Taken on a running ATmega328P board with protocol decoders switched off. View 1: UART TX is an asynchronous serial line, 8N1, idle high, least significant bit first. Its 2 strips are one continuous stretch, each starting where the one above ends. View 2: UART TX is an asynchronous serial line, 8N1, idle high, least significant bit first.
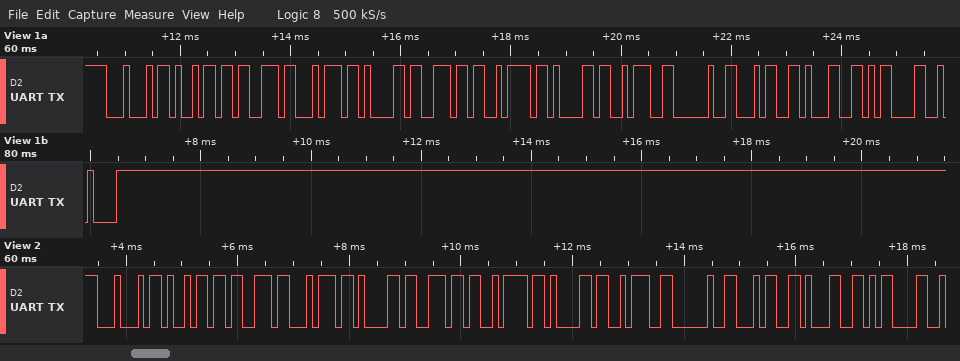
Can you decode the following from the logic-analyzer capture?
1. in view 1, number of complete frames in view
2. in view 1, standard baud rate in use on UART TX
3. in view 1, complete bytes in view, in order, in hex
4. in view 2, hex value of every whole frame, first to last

14
9600 baud
44 69 73 74 61 6E 7A 61 3A 20 34 31 0D 0A
0x44 0x69 0x73 0x74 0x61 0x6E 0x7A 0x61 0x3A 0x20 0x34 0x31 0x0D
